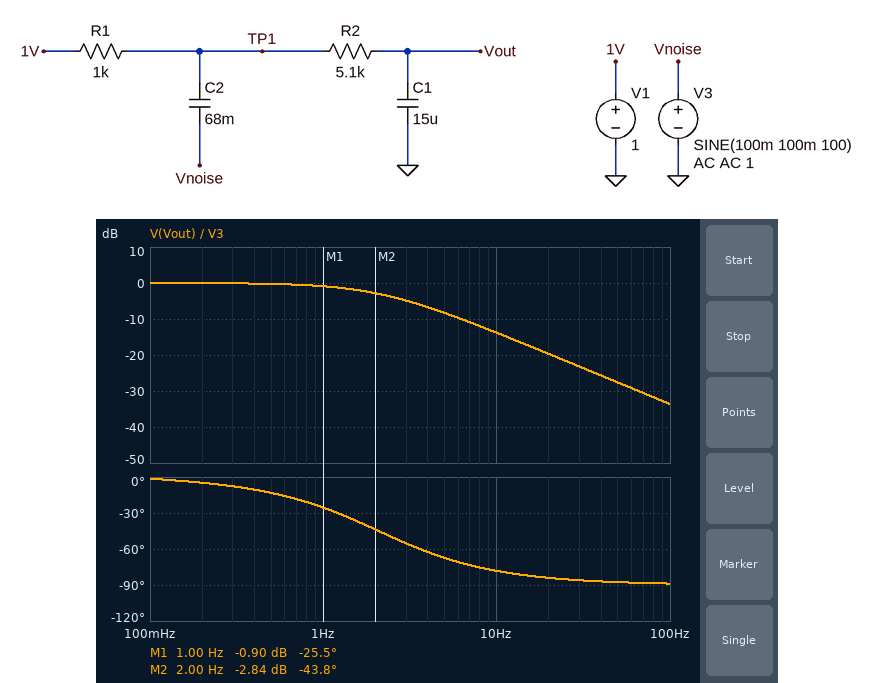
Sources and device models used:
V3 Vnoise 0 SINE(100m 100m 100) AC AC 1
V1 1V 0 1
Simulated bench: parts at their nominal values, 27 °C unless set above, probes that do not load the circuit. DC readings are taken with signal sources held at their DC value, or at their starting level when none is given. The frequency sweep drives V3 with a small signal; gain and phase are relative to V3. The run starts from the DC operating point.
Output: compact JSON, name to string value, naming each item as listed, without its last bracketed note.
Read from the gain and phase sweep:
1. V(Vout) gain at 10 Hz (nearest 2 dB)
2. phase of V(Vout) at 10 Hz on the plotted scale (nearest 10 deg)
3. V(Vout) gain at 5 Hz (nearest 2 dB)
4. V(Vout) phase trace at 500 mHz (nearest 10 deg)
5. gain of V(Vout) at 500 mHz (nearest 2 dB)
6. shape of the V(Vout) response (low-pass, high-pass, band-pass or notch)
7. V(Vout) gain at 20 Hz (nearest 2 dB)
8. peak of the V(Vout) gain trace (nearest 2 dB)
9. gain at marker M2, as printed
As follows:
{"V(Vout) gain at 10 Hz": "-14 dB", "phase of V(Vout) at 10 Hz on the plotted scale": "-80 deg", "V(Vout) gain at 5 Hz": "-8 dB", "V(Vout) phase trace at 500 mHz": "-10 deg", "gain of V(Vout) at 500 mHz": "0 dB", "shape of the V(Vout) response": "low-pass", "V(Vout) gain at 20 Hz": "-20 dB", "peak of the V(Vout) gain trace": "0 dB", "gain at marker M2, as printed": "-2.84 dB"}
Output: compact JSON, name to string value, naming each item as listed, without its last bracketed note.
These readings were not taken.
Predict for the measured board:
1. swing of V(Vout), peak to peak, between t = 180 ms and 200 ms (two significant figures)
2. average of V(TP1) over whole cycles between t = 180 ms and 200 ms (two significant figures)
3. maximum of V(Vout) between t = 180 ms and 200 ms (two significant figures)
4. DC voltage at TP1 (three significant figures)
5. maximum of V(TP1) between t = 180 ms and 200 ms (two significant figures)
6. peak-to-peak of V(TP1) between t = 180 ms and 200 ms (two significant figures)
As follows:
{"swing of V(Vout), peak to peak, between t = 180 ms and 200 ms": "4.2 mV", "average of V(TP1) over whole cycles between t = 180 ms and 200 ms": "1.0 V", "maximum of V(Vout) between t = 180 ms and 200 ms": "1.0 V", "DC voltage at TP1": "1.00 V", "maximum of V(TP1) between t = 180 ms and 200 ms": "1.1 V", "peak-to-peak of V(TP1) between t = 180 ms and 200 ms": "200 mV"}
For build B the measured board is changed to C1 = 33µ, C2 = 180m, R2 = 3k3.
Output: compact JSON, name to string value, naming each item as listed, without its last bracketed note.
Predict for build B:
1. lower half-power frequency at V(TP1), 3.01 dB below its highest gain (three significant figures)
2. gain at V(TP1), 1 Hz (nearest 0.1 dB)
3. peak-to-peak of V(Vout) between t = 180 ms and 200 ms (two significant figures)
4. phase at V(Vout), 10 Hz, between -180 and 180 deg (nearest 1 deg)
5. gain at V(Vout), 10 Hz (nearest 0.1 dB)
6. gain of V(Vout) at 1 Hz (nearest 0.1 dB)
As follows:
{"lower half-power frequency at V(TP1), 3.01 dB below its highest gain": "884 µHz", "gain at V(TP1), 1 Hz": "0 dB", "peak-to-peak of V(Vout) between t = 180 ms and 200 ms": "3.0 mV", "phase at V(Vout), 10 Hz, between -180 and 180 deg": "-82 deg", "gain at V(Vout), 10 Hz": "-16.8 dB", "gain of V(Vout) at 1 Hz": "-1.7 dB"}
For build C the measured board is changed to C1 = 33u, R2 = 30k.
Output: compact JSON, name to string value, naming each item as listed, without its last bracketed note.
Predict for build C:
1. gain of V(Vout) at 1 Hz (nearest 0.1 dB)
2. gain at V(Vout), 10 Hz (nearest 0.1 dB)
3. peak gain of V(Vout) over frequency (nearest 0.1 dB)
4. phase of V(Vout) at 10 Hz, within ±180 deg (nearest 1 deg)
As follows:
{"gain of V(Vout) at 1 Hz": "-16.0 dB", "gain at V(Vout), 10 Hz": "-35.9 dB", "peak gain of V(Vout) over frequency": "-0.1 dB", "phase of V(Vout) at 10 Hz, within ±180 deg": "-89 deg"}
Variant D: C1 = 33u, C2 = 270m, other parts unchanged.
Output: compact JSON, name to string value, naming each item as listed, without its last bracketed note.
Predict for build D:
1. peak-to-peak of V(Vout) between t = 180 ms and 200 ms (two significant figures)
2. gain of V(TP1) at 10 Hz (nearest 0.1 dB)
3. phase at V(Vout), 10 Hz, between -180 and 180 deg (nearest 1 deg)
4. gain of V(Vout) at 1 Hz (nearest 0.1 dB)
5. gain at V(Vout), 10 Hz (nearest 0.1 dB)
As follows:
{"peak-to-peak of V(Vout) between t = 180 ms and 200 ms": "1.9 mV", "gain of V(TP1) at 10 Hz": "0 dB", "phase at V(Vout), 10 Hz, between -180 and 180 deg": "-85 deg", "gain of V(Vout) at 1 Hz": "-3.3 dB", "gain at V(Vout), 10 Hz": "-20.5 dB"}
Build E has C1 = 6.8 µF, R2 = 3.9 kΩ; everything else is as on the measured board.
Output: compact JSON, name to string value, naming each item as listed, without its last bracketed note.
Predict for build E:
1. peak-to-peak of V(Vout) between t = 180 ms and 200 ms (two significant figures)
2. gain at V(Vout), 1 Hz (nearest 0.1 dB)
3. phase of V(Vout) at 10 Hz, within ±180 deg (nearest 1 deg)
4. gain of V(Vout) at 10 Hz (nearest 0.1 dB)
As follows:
{"peak-to-peak of V(Vout) between t = 180 ms and 200 ms": "12 mV", "gain at V(Vout), 1 Hz": "-0.1 dB", "phase of V(Vout) at 10 Hz, within ±180 deg": "-59 deg", "gain of V(Vout) at 10 Hz": "-5.8 dB"}
